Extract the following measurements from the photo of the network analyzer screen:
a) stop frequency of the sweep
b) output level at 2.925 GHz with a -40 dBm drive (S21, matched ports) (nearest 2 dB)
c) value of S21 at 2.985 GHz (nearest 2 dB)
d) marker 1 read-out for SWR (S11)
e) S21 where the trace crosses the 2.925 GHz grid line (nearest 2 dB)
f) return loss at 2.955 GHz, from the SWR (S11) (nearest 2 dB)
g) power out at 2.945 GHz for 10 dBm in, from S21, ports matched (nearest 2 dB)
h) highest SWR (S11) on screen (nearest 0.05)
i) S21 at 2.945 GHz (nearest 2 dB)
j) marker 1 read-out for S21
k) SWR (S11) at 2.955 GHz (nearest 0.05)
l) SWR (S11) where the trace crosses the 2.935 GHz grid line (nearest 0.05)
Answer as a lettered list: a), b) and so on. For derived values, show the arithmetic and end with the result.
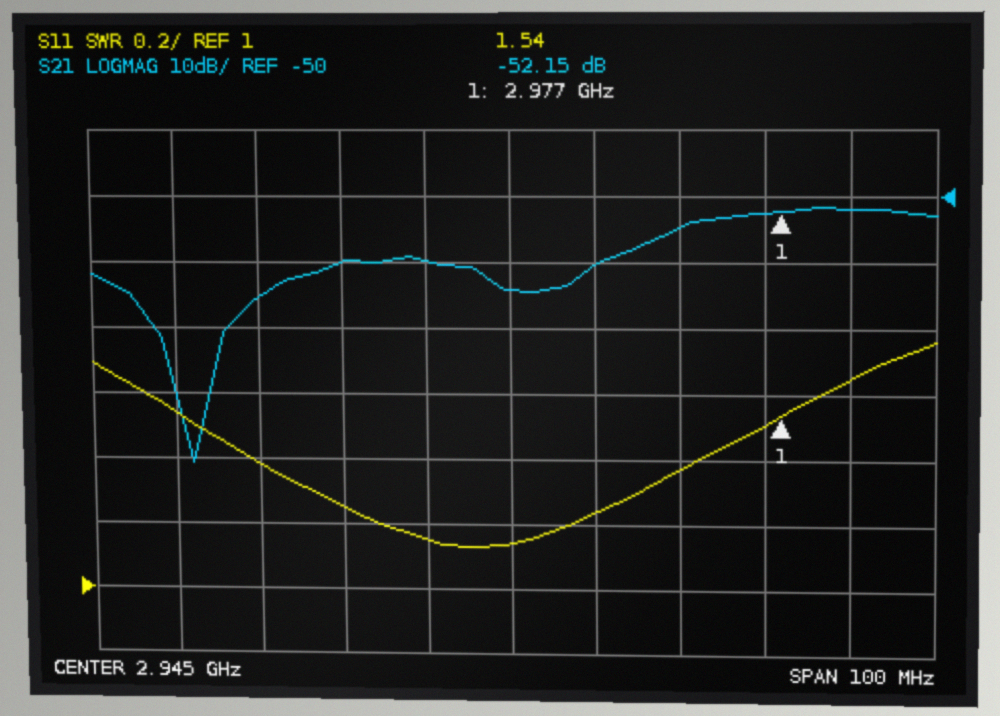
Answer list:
a) 2.995 GHz
b) -40 dBm + (-60 dB) = -100 dBm
c) -52 dB
d) 1.54
e) -60 dB
f) −20 log10((1.25 − 1)/(1.25 + 1)) ≈ 19.1 dB, so 20 dB to the nearest 2 dB
g) 10 dBm + (-64 dB) = -54 dBm
h) 1.75
i) -64 dB
j) -52.15 dB
k) 1.25
l) 1.15
